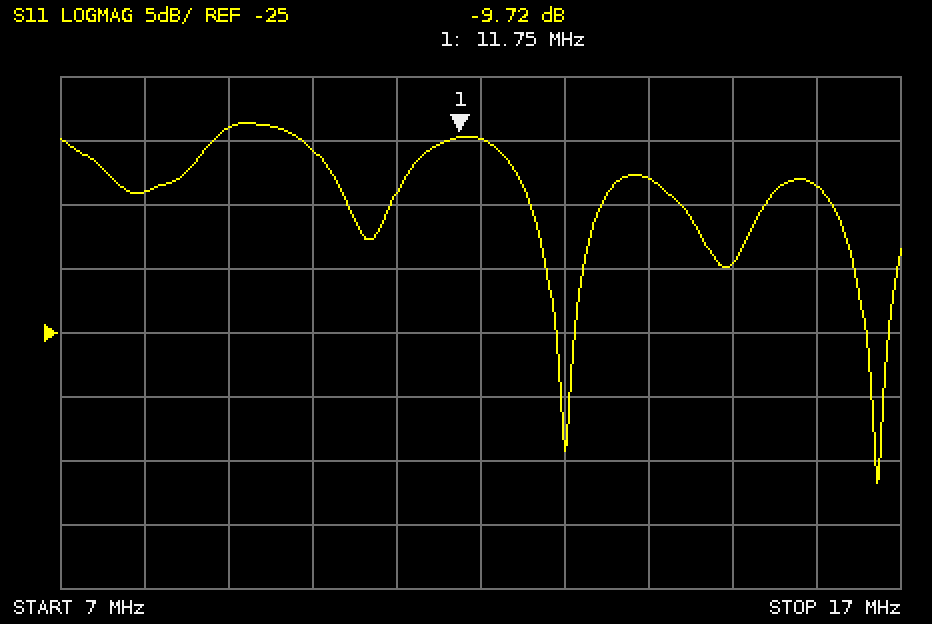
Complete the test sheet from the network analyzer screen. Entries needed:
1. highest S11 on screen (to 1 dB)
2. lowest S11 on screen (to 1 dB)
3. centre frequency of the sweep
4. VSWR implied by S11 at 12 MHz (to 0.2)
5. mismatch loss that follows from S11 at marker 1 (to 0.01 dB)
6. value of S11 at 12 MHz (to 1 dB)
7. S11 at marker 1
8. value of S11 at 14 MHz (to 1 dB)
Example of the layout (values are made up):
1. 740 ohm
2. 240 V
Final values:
1. -9 dB
2. -37 dB
3. 12 MHz
4. 2.0
5. 0.49 dB
6. -10 dB
7. -9.72 dB
8. -13 dB
